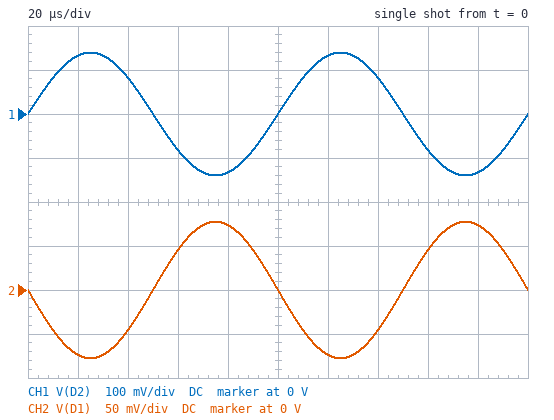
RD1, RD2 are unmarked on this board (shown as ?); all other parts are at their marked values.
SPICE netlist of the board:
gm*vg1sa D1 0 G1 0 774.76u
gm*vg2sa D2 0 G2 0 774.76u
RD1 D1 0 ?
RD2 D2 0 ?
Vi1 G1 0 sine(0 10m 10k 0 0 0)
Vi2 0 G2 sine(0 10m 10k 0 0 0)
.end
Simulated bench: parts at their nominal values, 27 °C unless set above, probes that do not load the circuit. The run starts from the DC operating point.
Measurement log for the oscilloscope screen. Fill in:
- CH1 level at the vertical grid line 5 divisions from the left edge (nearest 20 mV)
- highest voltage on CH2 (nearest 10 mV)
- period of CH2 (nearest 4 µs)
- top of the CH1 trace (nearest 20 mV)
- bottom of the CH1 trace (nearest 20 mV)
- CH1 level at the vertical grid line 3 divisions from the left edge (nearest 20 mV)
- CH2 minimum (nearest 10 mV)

0 V
80 mV
100 µs
140 mV
-140 mV
-80 mV
-80 mV
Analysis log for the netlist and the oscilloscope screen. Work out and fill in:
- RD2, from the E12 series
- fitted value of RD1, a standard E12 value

18 kΩ
10 kΩ
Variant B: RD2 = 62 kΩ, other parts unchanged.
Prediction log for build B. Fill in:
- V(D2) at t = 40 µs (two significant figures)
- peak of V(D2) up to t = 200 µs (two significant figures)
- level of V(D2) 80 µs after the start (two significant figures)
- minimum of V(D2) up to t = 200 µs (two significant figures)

280 mV
480 mV
-460 mV
-480 mV
